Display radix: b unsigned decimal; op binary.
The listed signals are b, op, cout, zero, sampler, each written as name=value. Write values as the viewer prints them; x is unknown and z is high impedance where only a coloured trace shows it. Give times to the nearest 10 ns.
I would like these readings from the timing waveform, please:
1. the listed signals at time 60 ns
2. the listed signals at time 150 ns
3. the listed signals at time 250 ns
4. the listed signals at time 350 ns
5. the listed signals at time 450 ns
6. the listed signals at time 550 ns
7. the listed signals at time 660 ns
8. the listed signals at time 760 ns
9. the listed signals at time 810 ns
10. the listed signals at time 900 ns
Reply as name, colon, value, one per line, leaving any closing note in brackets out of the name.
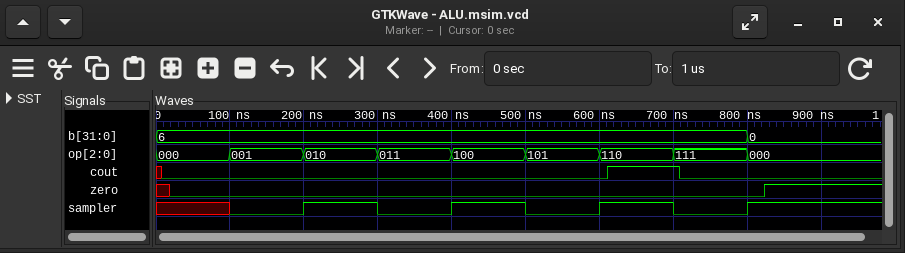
the listed signals at time 60 ns: b=6, op=000, cout=0, zero=0, sampler=x
the listed signals at time 150 ns: b=6, op=001, cout=0, zero=0, sampler=0
the listed signals at time 250 ns: b=6, op=010, cout=0, zero=0, sampler=1
the listed signals at time 350 ns: b=6, op=011, cout=0, zero=0, sampler=0
the listed signals at time 450 ns: b=6, op=100, cout=0, zero=0, sampler=1
the listed signals at time 550 ns: b=6, op=101, cout=0, zero=0, sampler=0
the listed signals at time 660 ns: b=6, op=110, cout=1, zero=0, sampler=1
the listed signals at time 760 ns: b=6, op=111, cout=0, zero=0, sampler=0
the listed signals at time 810 ns: b=0, op=000, cout=0, zero=0, sampler=1
the listed signals at time 900 ns: b=0, op=000, cout=0, zero=1, sampler=1
